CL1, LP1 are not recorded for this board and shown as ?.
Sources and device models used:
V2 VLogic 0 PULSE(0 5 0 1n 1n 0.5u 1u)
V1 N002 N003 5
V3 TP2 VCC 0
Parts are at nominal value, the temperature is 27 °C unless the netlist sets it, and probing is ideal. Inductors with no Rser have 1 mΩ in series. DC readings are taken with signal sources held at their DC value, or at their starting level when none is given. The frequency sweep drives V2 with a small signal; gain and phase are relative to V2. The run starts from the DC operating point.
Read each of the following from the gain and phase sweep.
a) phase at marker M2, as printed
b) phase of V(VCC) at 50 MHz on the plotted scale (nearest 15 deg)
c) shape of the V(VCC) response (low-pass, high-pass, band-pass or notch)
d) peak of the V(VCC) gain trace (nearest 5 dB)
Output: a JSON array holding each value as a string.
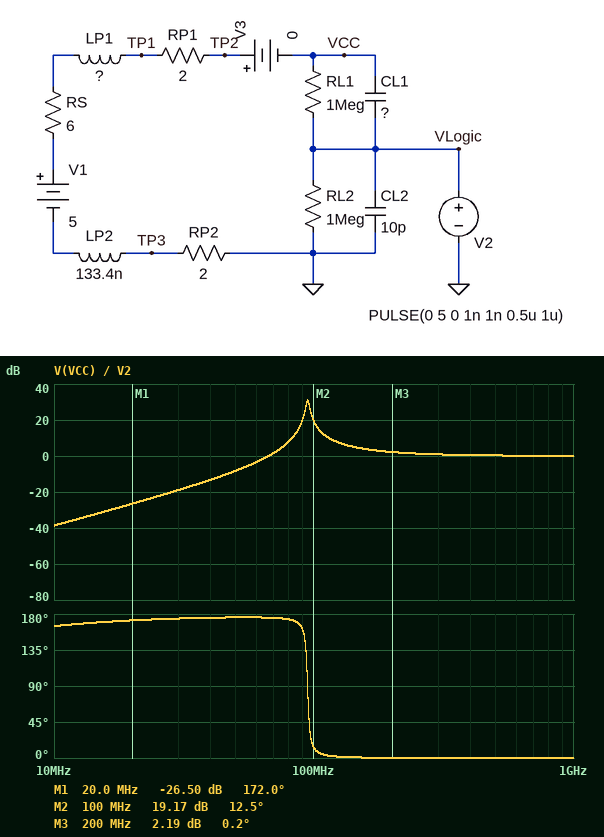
["12.5 deg", "180 deg", "high-pass", "30 dB"]
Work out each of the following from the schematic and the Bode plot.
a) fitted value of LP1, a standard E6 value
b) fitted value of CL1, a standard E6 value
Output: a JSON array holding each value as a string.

["470 nH", "4.7 pF"]
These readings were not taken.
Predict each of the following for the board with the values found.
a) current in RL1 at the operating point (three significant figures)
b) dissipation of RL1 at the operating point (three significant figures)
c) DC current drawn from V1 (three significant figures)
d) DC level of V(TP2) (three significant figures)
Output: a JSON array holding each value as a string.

["5.00 µA", "25.0 µW", "5.00 µA", "5.00 V"]
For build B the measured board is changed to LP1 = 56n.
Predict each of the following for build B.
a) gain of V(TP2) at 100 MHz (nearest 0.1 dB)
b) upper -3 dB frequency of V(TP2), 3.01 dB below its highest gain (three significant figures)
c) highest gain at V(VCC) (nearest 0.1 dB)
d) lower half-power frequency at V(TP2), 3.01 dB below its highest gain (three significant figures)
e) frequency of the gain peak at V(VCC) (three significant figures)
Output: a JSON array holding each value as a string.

["-5.3 dB", "173 MHz", "26.0 dB", "165 MHz", "169 MHz"]
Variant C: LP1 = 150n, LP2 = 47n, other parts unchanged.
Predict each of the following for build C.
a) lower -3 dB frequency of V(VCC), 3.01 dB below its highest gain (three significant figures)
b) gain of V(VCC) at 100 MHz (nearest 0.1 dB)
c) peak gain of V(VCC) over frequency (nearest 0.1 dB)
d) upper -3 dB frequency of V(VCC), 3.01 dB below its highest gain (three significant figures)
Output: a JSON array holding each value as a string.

["162 MHz", "-4.8 dB", "26.2 dB", "170 MHz"]
